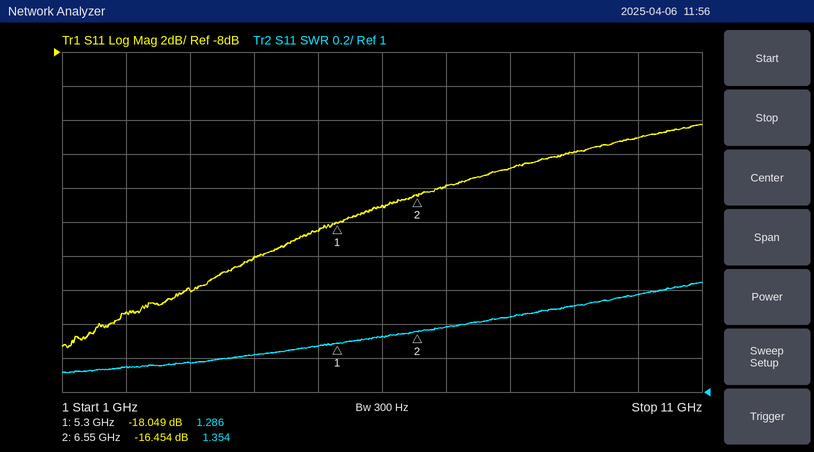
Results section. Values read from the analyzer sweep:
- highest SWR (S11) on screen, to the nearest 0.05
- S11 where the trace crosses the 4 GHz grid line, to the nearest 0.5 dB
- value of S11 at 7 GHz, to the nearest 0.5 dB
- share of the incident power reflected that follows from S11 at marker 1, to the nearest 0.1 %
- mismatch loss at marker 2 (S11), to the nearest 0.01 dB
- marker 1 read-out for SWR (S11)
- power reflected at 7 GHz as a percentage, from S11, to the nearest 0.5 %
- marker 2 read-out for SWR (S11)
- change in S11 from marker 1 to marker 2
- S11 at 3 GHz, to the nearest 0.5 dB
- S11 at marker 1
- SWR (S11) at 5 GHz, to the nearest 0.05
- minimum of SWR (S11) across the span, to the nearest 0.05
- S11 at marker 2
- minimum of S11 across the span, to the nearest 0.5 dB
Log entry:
1.65
-20.0 dB
-16.0 dB
1.6 %
0.10 dB
1.286
2.5 %
1.354
1.595 dB
-22.0 dB
-18.049 dB
1.25
1.10
-16.454 dB
-25.5 dB
